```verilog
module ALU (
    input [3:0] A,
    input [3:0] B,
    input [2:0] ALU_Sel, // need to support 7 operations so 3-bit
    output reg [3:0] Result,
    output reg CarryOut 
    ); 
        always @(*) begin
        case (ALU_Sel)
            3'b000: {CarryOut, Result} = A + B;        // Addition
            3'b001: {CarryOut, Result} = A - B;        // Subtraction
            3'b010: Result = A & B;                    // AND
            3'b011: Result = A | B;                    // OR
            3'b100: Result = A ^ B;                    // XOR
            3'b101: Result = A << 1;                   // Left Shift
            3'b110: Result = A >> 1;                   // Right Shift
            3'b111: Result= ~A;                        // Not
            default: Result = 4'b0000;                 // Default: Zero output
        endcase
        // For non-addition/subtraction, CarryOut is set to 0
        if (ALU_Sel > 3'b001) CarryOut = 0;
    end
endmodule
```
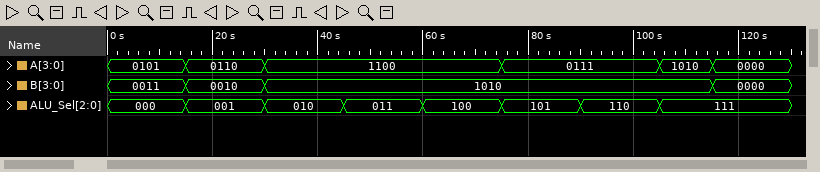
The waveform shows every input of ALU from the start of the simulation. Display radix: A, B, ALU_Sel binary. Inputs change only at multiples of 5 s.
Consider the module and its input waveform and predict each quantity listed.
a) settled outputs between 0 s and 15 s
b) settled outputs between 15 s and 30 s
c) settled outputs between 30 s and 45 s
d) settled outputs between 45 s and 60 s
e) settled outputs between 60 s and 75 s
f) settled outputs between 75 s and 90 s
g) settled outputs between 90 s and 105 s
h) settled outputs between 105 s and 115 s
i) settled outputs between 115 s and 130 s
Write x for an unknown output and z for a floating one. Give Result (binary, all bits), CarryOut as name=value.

Result=1000, CarryOut=0
Result=0100, CarryOut=0
Result=1000, CarryOut=0
Result=1110, CarryOut=0
Result=0110, CarryOut=0
Result=1110, CarryOut=0
Result=0011, CarryOut=0
Result=0101, CarryOut=0
Result=1111, CarryOut=0
